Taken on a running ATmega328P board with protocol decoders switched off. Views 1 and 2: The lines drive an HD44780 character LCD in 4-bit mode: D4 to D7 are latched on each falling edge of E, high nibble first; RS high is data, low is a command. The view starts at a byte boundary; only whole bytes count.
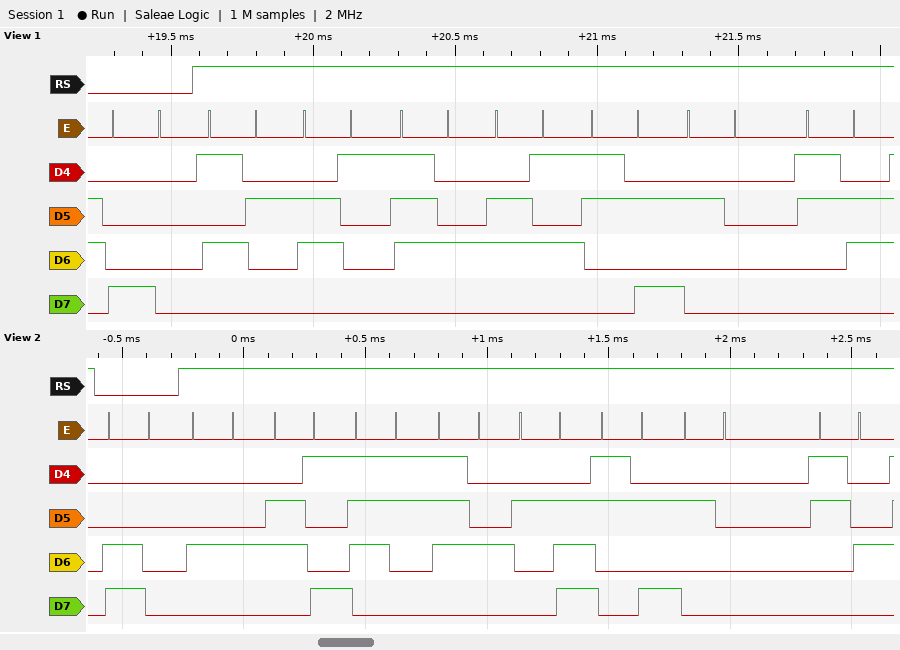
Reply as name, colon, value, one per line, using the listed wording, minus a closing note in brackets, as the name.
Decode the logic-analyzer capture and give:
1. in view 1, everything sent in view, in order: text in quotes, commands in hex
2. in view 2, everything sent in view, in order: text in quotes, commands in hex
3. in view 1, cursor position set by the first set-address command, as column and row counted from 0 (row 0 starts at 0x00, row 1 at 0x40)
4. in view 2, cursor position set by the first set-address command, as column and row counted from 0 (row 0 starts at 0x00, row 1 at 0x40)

in view 1, everything sent in view, in order: text in quotes, commands in hex: 0x80 "Rate: 6"
in view 2, everything sent in view, in order: text in quotes, commands in hex: 0xC0 "Dist.: 4"
in view 1, cursor position set by the first set-address command, as column and row counted from 0: column 0, row 0
in view 2, cursor position set by the first set-address command, as column and row counted from 0: column 0, row 1
